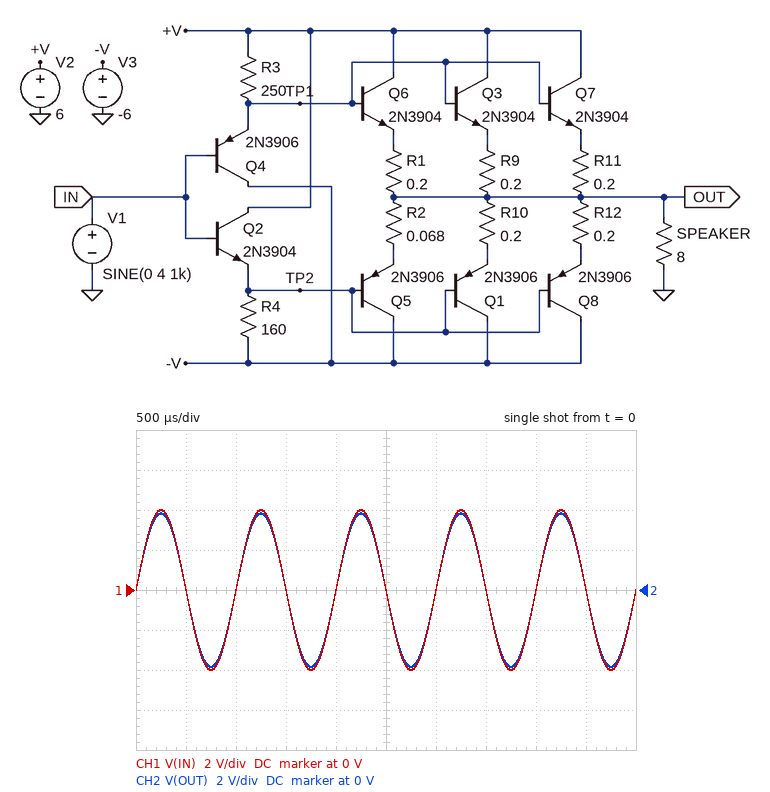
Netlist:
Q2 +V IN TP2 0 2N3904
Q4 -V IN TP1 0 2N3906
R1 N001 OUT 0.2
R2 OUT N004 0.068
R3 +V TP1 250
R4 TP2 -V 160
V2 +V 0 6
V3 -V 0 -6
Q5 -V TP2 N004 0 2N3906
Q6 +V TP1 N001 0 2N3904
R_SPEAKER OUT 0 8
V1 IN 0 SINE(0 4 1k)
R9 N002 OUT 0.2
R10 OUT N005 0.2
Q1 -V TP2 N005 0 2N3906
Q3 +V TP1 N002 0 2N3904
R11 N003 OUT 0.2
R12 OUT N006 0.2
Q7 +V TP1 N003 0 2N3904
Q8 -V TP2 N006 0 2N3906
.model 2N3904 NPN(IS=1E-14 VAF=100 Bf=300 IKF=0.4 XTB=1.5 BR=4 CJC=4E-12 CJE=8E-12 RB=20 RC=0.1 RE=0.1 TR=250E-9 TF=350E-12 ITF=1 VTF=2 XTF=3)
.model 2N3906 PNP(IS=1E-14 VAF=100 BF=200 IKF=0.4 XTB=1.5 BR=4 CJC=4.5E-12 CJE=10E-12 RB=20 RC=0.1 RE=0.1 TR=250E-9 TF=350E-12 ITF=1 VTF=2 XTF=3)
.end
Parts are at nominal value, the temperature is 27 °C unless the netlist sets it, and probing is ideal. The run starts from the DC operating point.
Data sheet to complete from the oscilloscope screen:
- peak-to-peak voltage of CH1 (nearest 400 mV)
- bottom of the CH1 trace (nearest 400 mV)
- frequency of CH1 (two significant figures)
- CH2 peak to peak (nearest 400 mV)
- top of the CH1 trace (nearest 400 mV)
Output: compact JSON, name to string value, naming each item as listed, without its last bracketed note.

{"peak-to-peak voltage of CH1": "8.0 V", "bottom of the CH1 trace": "-4.0 V", "frequency of CH1": "1.0 kHz", "CH2 peak to peak": "7.6 V", "top of the CH1 trace": "4.0 V"}
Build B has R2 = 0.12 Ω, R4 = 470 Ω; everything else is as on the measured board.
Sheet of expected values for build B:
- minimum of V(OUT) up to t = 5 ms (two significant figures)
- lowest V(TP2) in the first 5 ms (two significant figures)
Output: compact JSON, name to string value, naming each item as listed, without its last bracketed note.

{"minimum of V(OUT) up to t = 5 ms": "-3.7 V", "lowest V(TP2) in the first 5 ms": "-4.5 V"}
